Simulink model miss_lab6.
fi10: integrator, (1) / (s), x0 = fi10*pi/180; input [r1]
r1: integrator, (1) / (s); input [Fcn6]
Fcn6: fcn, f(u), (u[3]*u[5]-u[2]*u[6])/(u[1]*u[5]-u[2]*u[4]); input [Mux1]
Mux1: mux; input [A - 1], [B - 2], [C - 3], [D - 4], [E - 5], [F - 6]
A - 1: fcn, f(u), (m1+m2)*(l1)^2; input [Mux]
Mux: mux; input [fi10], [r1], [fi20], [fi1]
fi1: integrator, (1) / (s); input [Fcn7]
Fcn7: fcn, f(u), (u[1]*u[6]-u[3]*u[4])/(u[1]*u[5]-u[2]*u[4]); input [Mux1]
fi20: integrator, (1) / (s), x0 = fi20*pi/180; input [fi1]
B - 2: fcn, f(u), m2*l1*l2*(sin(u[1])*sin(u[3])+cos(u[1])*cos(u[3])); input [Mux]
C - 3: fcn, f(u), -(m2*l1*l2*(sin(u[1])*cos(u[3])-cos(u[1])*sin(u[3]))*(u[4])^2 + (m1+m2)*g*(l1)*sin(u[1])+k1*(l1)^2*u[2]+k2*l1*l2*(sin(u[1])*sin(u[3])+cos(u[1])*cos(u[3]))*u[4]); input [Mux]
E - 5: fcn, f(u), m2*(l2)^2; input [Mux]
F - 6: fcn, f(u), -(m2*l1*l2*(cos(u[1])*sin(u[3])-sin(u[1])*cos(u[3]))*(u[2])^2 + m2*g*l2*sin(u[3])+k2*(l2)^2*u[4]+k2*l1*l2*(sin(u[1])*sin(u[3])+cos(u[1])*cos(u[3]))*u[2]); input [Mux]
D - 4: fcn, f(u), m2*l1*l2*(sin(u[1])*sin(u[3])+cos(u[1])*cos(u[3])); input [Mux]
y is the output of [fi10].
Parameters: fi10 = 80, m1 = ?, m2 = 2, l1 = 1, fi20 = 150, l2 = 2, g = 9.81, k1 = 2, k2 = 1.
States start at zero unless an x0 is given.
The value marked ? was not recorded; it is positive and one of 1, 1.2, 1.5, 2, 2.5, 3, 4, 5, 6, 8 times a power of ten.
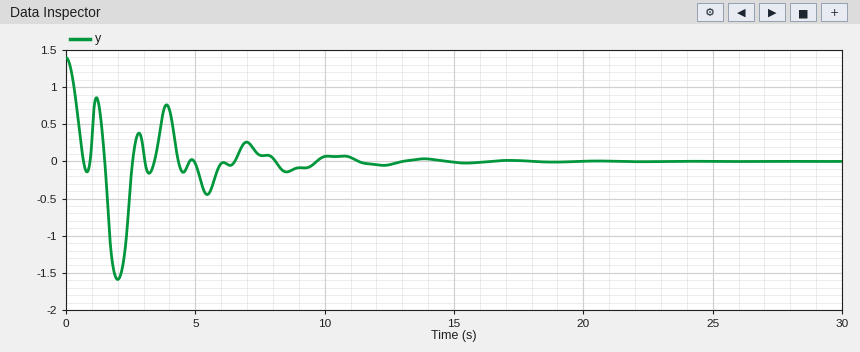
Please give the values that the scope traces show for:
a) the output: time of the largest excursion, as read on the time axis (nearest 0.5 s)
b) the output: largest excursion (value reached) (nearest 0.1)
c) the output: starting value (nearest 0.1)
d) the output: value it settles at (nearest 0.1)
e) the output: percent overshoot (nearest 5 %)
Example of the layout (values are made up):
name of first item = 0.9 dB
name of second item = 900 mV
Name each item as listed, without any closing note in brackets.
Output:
the output: time of the largest excursion, as read on the time axis = 2.0 s
the output: largest excursion (value reached) = -1.6
the output: starting value = 1.4
the output: value it settles at = 0.0
the output: percent overshoot = 115 %
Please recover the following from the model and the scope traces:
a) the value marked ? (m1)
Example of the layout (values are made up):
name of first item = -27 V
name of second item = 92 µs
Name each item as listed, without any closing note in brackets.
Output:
the value marked ? = 1
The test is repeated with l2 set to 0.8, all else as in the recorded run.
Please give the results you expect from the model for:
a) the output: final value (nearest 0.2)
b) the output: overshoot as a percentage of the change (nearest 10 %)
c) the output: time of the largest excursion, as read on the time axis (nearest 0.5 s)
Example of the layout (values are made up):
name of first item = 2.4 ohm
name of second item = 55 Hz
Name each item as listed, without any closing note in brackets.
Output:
the output: final value = 0.0
the output: overshoot as a percentage of the change = 90 %
the output: time of the largest excursion, as read on the time axis = 1.5 s
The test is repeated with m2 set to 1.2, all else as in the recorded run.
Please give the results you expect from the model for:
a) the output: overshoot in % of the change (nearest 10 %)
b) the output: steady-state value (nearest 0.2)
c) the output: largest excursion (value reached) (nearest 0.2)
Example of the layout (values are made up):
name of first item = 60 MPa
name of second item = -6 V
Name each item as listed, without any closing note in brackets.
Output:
the output: overshoot in % of the change = 70 %
the output: steady-state value = 0.0
the output: largest excursion (value reached) = -1.0
